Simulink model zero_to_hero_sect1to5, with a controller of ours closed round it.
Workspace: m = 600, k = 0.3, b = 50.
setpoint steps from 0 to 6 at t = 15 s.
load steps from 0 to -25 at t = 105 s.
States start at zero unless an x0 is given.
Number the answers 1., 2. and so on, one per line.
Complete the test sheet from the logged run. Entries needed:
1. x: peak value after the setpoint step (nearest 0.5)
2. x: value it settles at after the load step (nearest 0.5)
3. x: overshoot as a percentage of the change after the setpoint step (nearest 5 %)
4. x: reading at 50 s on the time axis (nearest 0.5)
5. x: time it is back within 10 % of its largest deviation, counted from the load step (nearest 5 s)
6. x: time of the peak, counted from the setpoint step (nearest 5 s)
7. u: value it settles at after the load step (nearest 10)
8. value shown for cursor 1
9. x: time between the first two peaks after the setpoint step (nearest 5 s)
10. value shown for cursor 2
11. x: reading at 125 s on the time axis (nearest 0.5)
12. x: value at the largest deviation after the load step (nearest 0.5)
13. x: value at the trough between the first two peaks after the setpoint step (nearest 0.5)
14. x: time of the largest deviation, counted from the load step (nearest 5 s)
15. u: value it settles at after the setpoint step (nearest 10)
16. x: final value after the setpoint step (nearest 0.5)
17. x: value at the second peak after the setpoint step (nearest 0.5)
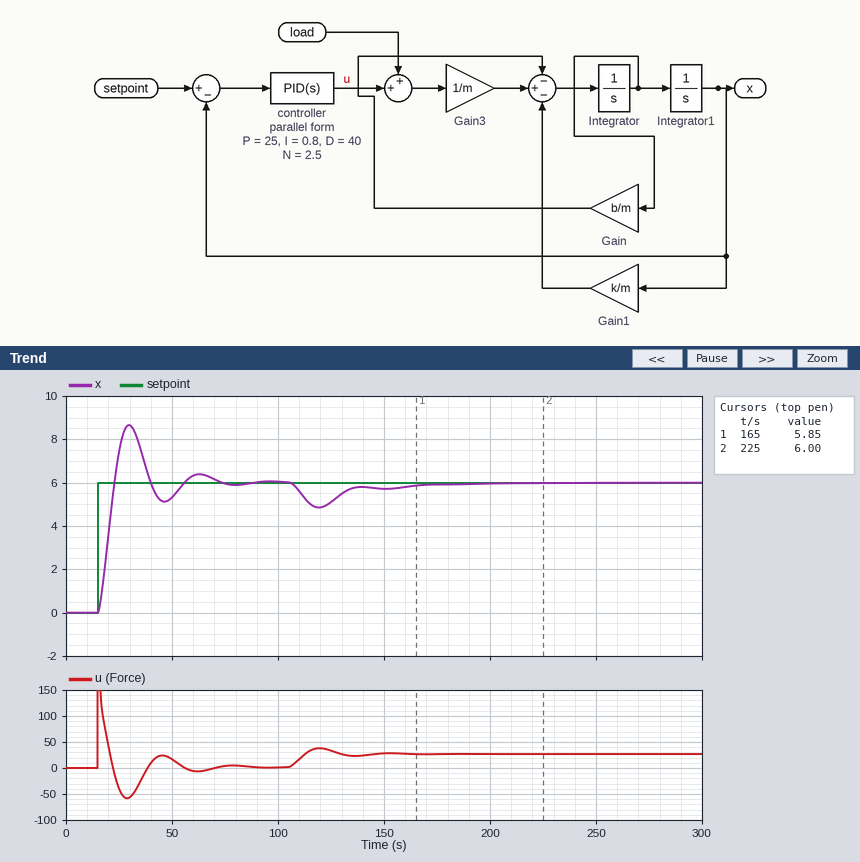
1. 8.5
2. 6.0
3. 45 %
4. 5.5
5. 60 s
6. 15 s
7. 30
8. 5.85
9. 35 s
10. 6.00
11. 5.0
12. 5.0
13. 5.0
14. 15 s
15. 0
16. 6.0
17. 6.5
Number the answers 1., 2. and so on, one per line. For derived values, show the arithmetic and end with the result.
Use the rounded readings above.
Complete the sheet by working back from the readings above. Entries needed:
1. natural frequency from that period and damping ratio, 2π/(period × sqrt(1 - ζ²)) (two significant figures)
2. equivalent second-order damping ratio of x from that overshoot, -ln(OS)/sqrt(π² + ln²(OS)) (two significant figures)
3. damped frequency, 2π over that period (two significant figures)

1. 2π / (35 × sqrt(1 - 0.25²)) = 0.19 rad/s
2. ln(0.45) = -0.799; 0.799 / sqrt(9.870 + 0.638) = 0.25
3. 2π / 35 = 0.18 rad/s
